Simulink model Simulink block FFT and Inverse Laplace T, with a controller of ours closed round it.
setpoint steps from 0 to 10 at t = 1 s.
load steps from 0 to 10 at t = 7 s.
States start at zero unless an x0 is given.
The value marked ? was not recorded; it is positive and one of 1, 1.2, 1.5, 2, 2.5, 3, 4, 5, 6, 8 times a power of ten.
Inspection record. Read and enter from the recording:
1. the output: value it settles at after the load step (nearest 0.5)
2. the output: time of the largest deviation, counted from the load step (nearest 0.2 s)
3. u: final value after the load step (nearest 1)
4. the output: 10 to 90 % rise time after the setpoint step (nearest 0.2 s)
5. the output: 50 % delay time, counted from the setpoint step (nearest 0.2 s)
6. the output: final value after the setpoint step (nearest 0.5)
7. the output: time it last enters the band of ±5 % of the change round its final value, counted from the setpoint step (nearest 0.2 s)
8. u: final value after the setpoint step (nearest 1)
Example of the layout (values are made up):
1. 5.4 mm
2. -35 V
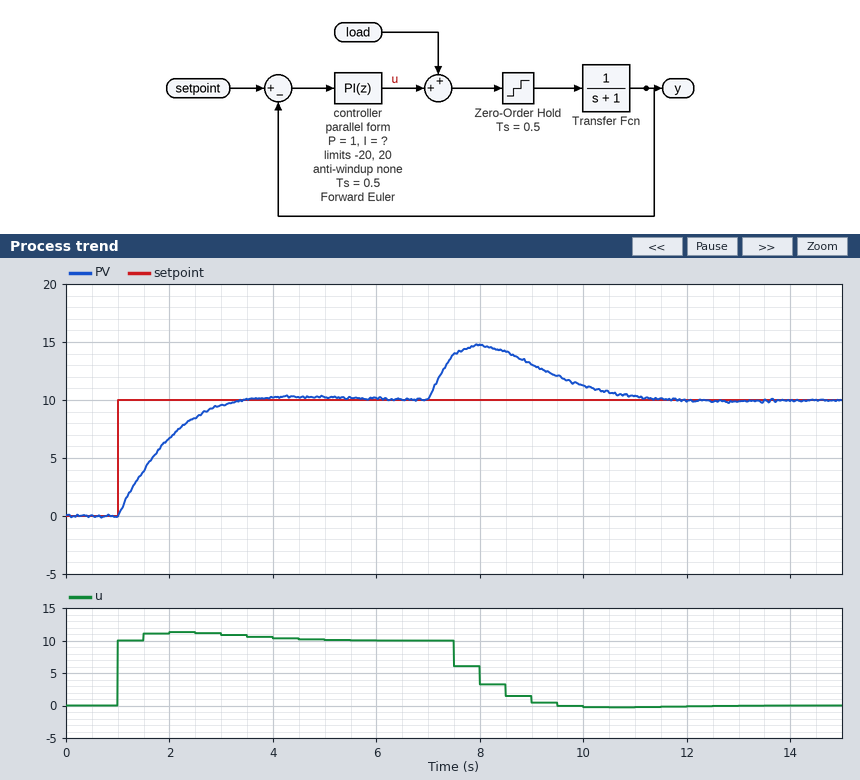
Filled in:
1. 10.0
2. 1.0 s
3. 0
4. 1.6 s
5. 0.6 s
6. 10.0
7. 2.0 s
8. 10
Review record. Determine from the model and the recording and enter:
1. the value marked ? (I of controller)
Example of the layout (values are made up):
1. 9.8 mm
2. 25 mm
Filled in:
1. 1
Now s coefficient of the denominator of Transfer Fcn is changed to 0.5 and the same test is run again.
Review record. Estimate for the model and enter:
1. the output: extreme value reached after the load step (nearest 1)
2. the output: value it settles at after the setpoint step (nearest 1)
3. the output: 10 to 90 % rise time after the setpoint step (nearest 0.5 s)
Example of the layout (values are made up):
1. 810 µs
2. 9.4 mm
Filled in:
1. 16
2. 10
3. 2.0 s
